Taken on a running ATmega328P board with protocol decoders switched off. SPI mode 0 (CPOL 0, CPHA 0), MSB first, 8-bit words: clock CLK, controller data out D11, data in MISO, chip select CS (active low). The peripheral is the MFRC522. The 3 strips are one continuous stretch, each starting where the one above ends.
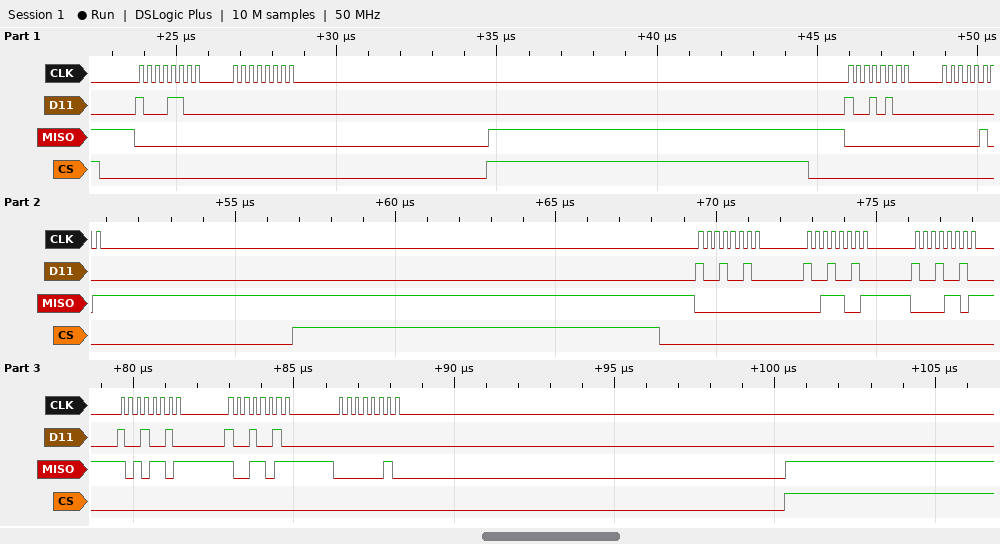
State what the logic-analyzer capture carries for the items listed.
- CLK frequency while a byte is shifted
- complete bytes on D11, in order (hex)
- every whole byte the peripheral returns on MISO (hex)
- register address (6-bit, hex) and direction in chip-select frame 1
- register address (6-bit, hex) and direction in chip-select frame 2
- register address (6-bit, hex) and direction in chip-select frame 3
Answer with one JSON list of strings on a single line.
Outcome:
["4 MHz", "8C 00 94 00 92 92 92 92 92 00", "00 00 00 05 00 39 0D AD 9B 02", "0x06 read", "0x0A read", "0x09 read"]
